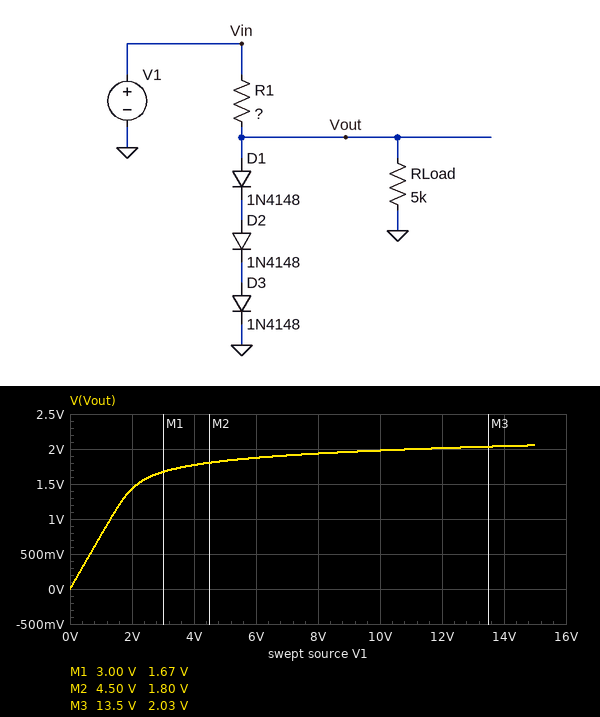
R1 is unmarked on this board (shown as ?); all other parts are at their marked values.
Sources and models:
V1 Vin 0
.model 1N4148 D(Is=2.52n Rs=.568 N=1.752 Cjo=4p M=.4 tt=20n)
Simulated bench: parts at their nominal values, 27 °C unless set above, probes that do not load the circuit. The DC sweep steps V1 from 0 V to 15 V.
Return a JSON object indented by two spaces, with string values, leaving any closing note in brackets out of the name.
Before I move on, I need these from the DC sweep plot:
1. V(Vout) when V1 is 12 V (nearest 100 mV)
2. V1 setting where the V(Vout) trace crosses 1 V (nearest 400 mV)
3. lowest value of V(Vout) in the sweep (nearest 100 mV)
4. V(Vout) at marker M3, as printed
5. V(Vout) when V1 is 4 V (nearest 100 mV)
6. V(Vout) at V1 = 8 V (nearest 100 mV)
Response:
{
  "V(Vout) when V1 is 12 V": "2.0 V",
  "V1 setting where the V(Vout) trace crosses 1 V": "1.2 V",
  "lowest value of V(Vout) in the sweep": "0 V",
  "V(Vout) at marker M3, as printed": "2.03 V",
  "V(Vout) when V1 is 4 V": "1.8 V",
  "V(Vout) at V1 = 8 V": "1.9 V"
}
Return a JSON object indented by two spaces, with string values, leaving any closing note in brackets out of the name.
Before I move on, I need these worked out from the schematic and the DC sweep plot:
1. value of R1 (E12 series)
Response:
{
  "value of R1": "1.5 kΩ"
}
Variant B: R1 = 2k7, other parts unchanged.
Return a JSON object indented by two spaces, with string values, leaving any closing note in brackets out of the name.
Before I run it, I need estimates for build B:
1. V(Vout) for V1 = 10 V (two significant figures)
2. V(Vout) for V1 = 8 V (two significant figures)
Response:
{
  "V(Vout) for V1 = 10 V": "1.9 V",
  "V(Vout) for V1 = 8 V": "1.8 V"
}
